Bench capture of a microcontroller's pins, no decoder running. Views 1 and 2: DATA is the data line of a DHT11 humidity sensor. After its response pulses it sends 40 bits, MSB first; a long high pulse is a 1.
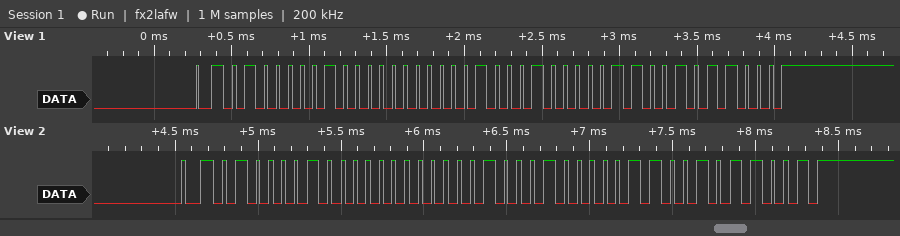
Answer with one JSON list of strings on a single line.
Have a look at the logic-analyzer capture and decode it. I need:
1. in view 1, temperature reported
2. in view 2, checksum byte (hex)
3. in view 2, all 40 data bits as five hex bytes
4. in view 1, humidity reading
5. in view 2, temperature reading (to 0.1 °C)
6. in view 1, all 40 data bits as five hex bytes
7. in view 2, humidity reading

["17.6 °C", "0x59", "42 00 11 06 59", "65 %", "17.6 °C", "41 00 11 06 58", "66 %"]
